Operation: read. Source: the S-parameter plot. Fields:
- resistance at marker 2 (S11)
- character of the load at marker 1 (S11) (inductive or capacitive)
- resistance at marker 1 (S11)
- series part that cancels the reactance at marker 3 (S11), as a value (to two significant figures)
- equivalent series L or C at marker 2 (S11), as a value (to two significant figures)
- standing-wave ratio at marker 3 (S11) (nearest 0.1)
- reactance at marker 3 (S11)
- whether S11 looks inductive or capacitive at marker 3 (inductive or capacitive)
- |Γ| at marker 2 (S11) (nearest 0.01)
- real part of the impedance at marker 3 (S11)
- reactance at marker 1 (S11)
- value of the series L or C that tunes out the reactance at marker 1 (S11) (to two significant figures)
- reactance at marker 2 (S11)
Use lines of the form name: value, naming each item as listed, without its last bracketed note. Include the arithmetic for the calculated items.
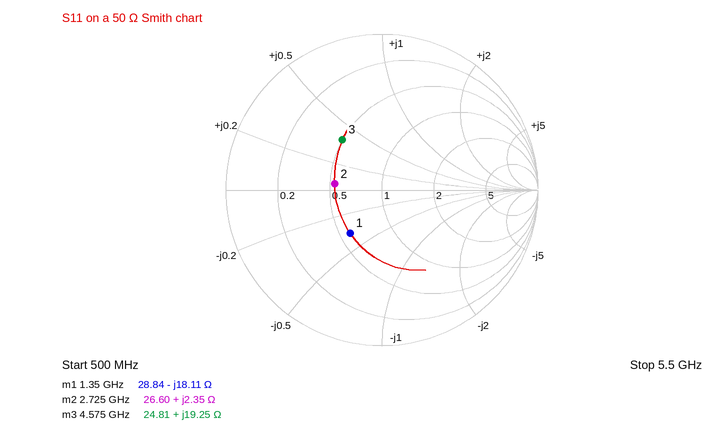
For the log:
resistance at marker 2: 26.60 Ω
character of the load at marker 1 (S11): capacitive
resistance at marker 1: 28.84 Ω
series part that cancels the reactance at marker 3 (S11), as a value: C = 1/(2π × 4.575 GHz × 19.25 Ω) ≈ 1.8 pF
equivalent series L or C at marker 2 (S11), as a value: L = 2.35 Ω/(2π × 2.725 GHz) ≈ 137 pH, so 140 pH to two significant figures
standing-wave ratio at marker 3 (S11): 2.4
reactance at marker 3: +19.25 Ω
whether S11 looks inductive or capacitive at marker 3: inductive
|Γ| at marker 2 (S11): 0.31
real part of the impedance at marker 3: 24.81 Ω
reactance at marker 1: -18.11 Ω
value of the series L or C that tunes out the reactance at marker 1 (S11): L = 18.11 Ω/(2π × 1.35 GHz) ≈ 2.1 nH
reactance at marker 2: +2.35 Ω
